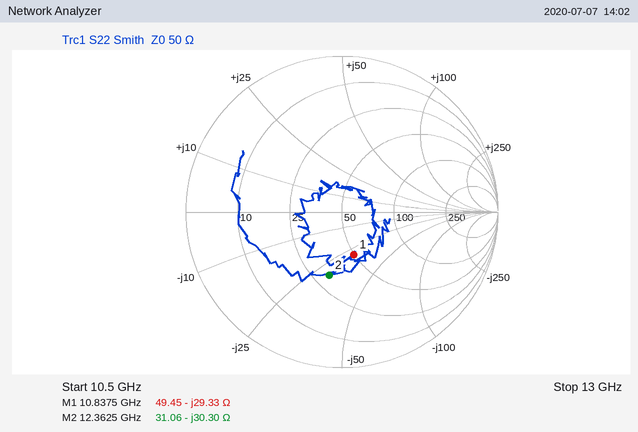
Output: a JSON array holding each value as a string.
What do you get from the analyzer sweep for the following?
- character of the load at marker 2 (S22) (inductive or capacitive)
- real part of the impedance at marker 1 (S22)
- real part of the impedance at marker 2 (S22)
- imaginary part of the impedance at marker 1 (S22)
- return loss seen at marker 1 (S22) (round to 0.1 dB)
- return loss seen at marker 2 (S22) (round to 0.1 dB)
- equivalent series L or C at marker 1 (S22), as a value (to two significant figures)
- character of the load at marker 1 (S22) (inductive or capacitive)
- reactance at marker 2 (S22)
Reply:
["capacitive", "49.45 Ω", "31.06 Ω", "-29.33 Ω", "11.0 dB", "7.7 dB", "500 fF", "capacitive", "-30.30 Ω"]
